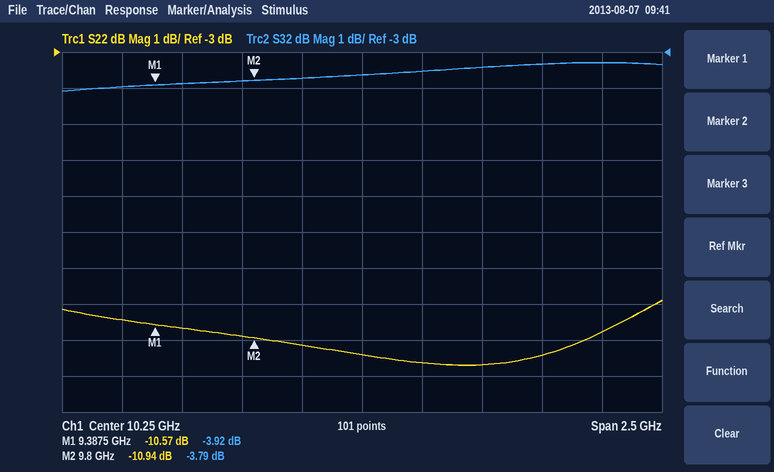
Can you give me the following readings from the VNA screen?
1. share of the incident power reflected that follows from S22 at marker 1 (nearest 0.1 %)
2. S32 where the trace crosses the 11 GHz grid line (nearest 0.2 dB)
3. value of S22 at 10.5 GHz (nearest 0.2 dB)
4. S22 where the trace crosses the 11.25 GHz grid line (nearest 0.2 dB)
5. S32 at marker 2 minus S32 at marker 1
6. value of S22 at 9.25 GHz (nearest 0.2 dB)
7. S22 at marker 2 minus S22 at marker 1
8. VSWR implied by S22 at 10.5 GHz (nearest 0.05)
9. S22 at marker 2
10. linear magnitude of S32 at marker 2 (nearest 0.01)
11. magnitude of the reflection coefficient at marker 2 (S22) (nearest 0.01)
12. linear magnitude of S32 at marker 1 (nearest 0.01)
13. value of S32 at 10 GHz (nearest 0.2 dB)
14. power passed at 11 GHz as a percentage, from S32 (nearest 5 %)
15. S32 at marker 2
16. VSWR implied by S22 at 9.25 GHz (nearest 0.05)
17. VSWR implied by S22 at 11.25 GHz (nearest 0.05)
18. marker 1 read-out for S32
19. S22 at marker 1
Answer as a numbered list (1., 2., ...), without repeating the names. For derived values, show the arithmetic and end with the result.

1. 10^(-10.57/10) ≈ 8.8 %
2. -3.4 dB
3. -11.6 dB
4. -10.8 dB
5. -3.79 − (-3.92) = 0.13 dB
6. -10.4 dB
7. -10.94 − (-10.57) = -0.37 dB
8. |Γ| = 10^(-11.6/20) = 0.2630; VSWR = (1 + 0.2630)/(1 − 0.2630) ≈ 1.71, so 1.70 to the nearest 0.05
9. -10.94 dB
10. 10^(-3.79/20) ≈ 0.65
11. 10^(-10.94/20) ≈ 0.28
12. 10^(-3.92/20) ≈ 0.64
13. -3.8 dB
14. 10^(-3.4/10) ≈ 45.7 %, so 45 % to the nearest 5 %
15. -3.79 dB
16. |Γ| = 10^(-10.4/20) = 0.3020; VSWR = (1 + 0.3020)/(1 − 0.3020) ≈ 1.87, so 1.85 to the nearest 0.05
17. |Γ| = 10^(-10.8/20) = 0.2884; VSWR = (1 + 0.2884)/(1 − 0.2884) ≈ 1.81, so 1.80 to the nearest 0.05
18. -3.92 dB
19. -10.57 dB
